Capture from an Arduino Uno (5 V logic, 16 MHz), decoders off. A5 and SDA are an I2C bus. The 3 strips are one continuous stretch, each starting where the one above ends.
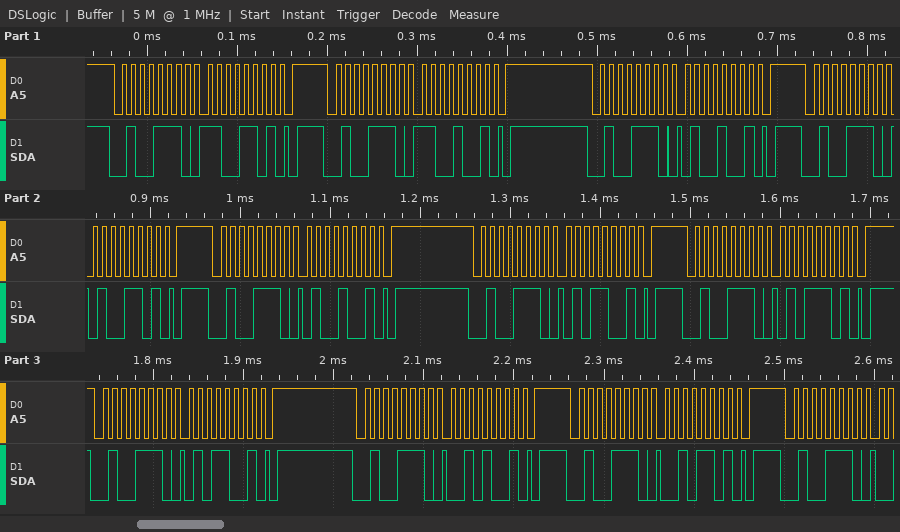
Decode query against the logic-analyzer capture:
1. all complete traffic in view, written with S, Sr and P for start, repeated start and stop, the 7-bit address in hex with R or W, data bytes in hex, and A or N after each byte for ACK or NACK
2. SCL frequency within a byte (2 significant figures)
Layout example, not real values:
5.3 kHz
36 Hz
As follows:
S 27W A CD A P S 27W A C9 A P S 27W A 49 A P S 27W A 4D A P S 27W A 49 A P S 27W A 59 A P S 27W A 5D A P S 27W A 59 A P S 27W A 29 A P S 27W A 2D A P S 27W A
100 kHz
